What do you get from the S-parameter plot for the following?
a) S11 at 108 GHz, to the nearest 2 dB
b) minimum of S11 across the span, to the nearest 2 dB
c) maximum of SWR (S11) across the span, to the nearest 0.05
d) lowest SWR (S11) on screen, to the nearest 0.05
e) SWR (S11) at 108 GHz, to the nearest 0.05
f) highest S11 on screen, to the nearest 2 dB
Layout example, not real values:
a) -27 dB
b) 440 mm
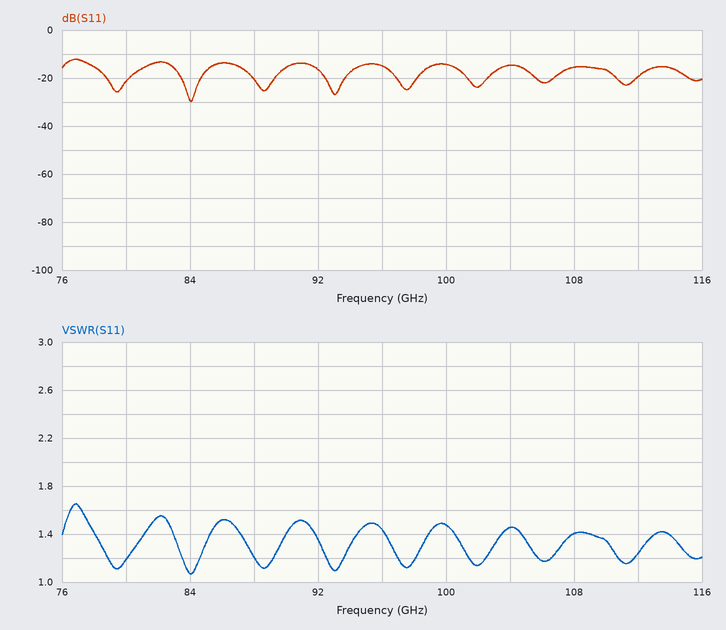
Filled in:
a) -16 dB
b) -30 dB
c) 1.65
d) 1.05
e) 1.40
f) -12 dB
